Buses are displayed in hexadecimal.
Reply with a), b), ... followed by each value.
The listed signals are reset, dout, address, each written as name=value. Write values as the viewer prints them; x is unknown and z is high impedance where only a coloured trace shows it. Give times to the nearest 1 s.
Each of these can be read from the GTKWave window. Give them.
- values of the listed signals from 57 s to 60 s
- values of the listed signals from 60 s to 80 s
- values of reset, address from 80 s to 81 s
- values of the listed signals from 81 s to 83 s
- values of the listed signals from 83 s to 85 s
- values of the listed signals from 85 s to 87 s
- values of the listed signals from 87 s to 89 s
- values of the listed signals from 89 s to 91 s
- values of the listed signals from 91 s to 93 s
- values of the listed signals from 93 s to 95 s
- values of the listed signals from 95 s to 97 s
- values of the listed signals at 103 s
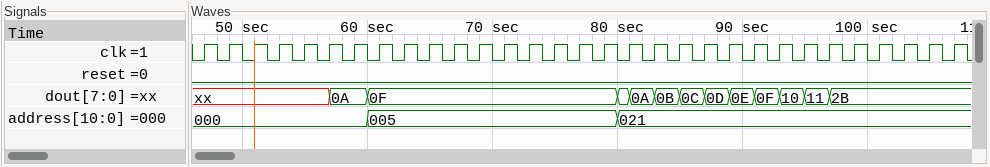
a) reset=0, dout=0A, address=000
b) reset=0, dout=0F, address=005
c) reset=0, address=021
d) reset=0, dout=0A, address=021
e) reset=0, dout=0B, address=021
f) reset=0, dout=0C, address=021
g) reset=0, dout=0D, address=021
h) reset=0, dout=0E, address=021
i) reset=0, dout=0F, address=021
j) reset=0, dout=10, address=021
k) reset=0, dout=11, address=021
l) reset=0, dout=2B, address=021
